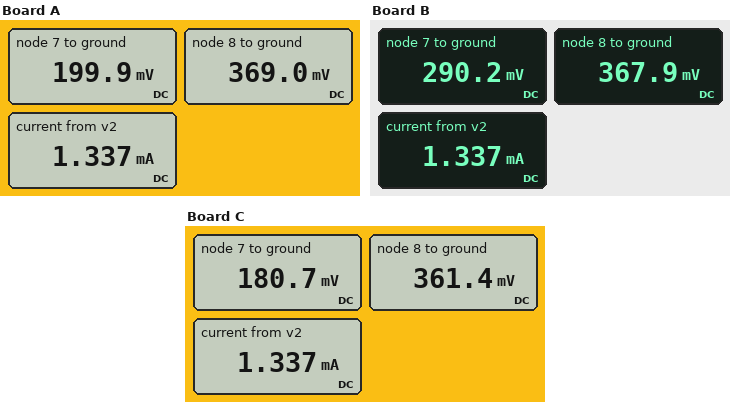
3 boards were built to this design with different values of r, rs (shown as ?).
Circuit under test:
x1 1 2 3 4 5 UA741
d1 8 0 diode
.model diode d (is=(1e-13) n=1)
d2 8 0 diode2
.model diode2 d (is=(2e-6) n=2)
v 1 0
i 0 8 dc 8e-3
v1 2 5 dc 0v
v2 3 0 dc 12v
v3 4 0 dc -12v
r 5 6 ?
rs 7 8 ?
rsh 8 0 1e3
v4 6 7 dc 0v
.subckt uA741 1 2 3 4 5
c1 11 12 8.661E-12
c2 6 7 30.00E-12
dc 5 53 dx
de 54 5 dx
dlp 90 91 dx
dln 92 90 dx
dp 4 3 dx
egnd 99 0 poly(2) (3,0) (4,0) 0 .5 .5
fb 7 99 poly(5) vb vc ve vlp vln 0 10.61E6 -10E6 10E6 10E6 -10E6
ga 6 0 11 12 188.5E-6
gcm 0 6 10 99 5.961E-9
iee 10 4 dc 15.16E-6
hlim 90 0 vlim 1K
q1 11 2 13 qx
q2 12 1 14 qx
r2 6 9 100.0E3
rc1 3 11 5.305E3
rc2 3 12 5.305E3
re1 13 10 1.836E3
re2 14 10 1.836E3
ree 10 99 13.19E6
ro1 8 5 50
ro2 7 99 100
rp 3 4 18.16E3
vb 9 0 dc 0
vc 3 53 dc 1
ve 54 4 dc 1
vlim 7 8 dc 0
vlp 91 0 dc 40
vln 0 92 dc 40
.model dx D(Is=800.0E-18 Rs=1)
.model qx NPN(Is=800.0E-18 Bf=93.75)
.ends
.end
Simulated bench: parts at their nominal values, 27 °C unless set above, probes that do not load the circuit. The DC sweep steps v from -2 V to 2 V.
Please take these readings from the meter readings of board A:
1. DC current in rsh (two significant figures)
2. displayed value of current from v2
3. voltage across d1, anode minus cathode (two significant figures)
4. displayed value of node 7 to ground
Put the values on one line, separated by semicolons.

370 µA; 1.337 mA; 370 mV; 199.9 mV
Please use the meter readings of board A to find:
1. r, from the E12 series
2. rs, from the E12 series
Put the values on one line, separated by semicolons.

39 Ω; 33 Ω
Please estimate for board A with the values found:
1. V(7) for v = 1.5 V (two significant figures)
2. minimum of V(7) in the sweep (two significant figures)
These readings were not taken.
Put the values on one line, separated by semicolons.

950 mV; -1.6 V
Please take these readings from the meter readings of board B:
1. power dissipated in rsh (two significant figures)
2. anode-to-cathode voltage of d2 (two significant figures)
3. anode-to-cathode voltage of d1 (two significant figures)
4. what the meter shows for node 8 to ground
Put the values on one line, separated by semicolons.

140 µW; 370 mV; 370 mV; 367.9 mV
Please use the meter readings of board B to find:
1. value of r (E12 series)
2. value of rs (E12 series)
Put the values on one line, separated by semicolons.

56 Ω; 15 Ω
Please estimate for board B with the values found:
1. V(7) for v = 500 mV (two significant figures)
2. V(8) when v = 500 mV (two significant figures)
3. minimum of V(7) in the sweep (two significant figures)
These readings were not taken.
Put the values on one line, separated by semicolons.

450 mV; 430 mV; -1.5 V
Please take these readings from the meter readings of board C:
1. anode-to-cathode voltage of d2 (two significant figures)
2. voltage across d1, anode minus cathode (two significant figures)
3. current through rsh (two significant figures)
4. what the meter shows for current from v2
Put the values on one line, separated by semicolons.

360 mV; 360 mV; 360 µA; 1.337 mA
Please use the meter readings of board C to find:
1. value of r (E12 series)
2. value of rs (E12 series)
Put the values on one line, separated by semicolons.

33 Ω; 33 Ω
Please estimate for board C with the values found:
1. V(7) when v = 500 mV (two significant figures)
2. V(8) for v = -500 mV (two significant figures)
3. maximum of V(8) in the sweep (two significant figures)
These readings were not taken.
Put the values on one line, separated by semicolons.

470 mV; 26 mV; 500 mV
